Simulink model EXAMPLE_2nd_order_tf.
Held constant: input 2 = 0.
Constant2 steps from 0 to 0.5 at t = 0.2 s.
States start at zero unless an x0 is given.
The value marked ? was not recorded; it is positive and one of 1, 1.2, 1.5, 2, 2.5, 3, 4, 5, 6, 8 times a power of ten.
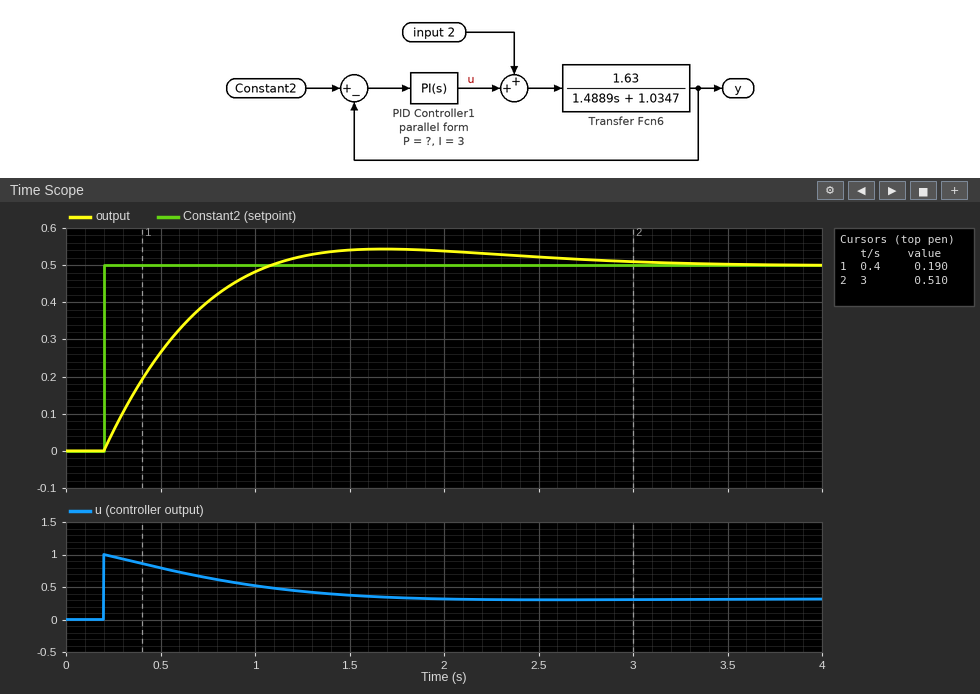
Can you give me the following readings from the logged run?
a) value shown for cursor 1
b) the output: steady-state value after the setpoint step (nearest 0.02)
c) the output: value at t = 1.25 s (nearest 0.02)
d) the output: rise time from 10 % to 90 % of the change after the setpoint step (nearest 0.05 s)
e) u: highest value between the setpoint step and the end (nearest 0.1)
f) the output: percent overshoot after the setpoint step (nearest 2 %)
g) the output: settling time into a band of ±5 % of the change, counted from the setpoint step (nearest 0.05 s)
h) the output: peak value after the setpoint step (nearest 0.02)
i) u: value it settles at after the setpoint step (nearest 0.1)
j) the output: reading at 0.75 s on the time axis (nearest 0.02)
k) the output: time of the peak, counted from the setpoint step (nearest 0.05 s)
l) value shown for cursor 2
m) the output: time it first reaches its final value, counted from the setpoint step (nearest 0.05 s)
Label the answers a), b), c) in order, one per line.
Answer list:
a) 0.190
b) 0.50
c) 0.52
d) 0.65 s
e) 1.0
f) 8 %
g) 2.20 s
h) 0.54
i) 0.3
j) 0.40
k) 1.50 s
l) 0.510
m) 0.90 s
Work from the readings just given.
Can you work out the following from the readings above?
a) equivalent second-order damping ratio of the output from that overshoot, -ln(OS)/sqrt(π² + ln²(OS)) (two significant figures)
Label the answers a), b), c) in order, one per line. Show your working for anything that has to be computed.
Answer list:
a) ln(0.08) = -2.526; 2.526 / sqrt(9.870 + 6.379) = 0.63
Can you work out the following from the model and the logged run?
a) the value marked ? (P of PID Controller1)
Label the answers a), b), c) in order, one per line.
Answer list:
a) 2
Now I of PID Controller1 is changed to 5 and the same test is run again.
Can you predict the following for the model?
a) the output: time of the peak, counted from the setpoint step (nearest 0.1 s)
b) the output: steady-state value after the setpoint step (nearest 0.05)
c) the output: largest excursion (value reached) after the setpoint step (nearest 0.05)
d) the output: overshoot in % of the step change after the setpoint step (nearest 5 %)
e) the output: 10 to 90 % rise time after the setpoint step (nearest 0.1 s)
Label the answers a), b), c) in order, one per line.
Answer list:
a) 1.1 s
b) 0.50
c) 0.60
d) 15 %
e) 0.5 s
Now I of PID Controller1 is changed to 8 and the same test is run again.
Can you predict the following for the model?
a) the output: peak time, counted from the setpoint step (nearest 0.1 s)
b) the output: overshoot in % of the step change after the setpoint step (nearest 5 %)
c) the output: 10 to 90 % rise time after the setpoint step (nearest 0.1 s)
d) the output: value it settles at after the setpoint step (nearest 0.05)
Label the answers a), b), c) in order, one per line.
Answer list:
a) 0.9 s
b) 25 %
c) 0.4 s
d) 0.50
